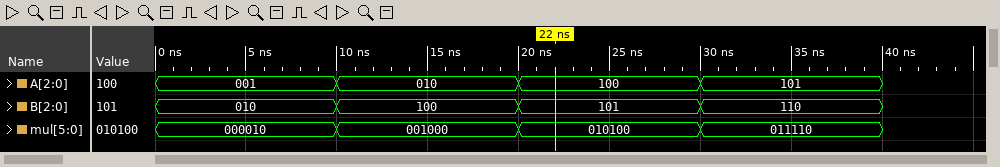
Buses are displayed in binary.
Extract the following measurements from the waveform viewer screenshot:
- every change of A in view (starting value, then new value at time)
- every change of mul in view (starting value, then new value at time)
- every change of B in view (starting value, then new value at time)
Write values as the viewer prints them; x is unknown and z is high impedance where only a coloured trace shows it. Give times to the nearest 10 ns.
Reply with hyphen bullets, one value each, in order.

- 001, 010 at 10 ns, 100 at 20 ns, 101 at 30 ns
- 000010, 001000 at 10 ns, 010100 at 20 ns, 011110 at 30 ns
- 010, 100 at 10 ns, 101 at 20 ns, 110 at 30 ns
